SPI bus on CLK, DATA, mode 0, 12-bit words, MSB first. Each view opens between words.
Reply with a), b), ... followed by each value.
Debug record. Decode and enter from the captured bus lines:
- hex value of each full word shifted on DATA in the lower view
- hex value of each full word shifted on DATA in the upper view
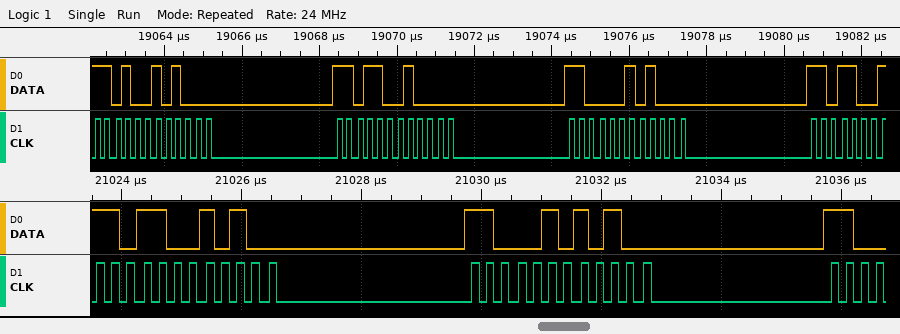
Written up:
a) D94, C54
b) D28, D90, C28
